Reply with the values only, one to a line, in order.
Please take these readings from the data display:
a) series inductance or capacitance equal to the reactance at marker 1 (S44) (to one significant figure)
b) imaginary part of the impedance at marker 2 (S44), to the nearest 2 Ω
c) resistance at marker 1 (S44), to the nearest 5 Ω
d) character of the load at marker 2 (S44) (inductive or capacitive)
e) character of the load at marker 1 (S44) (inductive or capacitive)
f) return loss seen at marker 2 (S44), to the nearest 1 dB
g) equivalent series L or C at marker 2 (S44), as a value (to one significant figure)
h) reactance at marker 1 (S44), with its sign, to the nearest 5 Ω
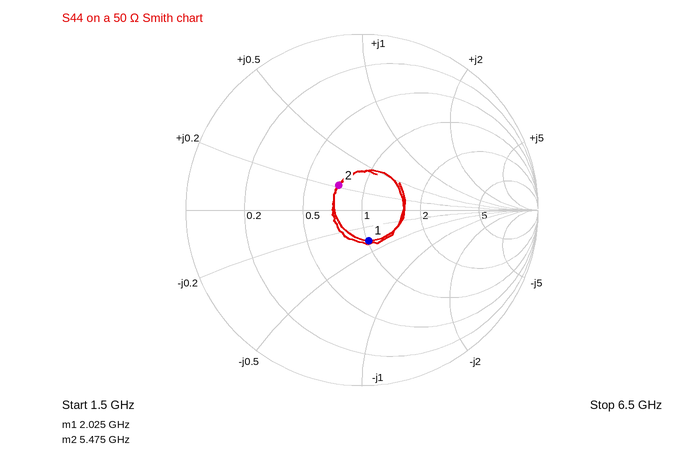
4 pF
+10 Ω
50 Ω
inductive
capacitive
14 dB
300 pH
-20 Ω
